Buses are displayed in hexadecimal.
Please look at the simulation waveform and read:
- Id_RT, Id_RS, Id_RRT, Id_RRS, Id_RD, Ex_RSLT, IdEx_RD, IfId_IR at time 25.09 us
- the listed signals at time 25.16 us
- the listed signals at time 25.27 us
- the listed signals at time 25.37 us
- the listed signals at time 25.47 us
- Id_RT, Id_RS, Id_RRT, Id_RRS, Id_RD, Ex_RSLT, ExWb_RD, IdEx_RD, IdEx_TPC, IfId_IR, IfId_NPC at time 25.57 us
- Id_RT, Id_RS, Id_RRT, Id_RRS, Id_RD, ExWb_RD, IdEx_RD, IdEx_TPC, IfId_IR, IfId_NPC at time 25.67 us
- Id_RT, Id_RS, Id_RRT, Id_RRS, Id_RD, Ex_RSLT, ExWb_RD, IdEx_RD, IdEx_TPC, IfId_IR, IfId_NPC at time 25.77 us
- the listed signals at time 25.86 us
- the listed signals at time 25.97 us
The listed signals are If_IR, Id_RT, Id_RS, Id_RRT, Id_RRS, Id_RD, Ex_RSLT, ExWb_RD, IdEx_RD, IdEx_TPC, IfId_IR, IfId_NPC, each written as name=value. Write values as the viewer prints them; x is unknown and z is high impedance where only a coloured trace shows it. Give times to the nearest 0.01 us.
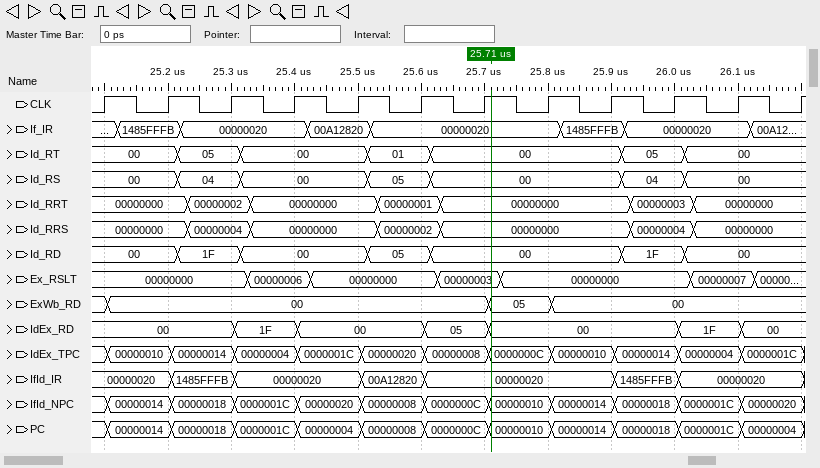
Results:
Id_RT=00, Id_RS=00, Id_RRT=00000000, Id_RRS=00000000, Id_RD=00, Ex_RSLT=00000000, IdEx_RD=00, IfId_IR=00000020
If_IR=1485FFFB, Id_RT=00, Id_RS=00, Id_RRT=00000000, Id_RRS=00000000, Id_RD=00, Ex_RSLT=00000000, ExWb_RD=00, IdEx_RD=00, IdEx_TPC=00000010, IfId_IR=00000020, IfId_NPC=00000014
If_IR=00000020, Id_RT=05, Id_RS=04, Id_RRT=00000002, Id_RRS=00000004, Id_RD=1F, Ex_RSLT=00000000, ExWb_RD=00, IdEx_RD=00, IdEx_TPC=00000014, IfId_IR=1485FFFB, IfId_NPC=00000018
If_IR=00000020, Id_RT=00, Id_RS=00, Id_RRT=00000000, Id_RRS=00000000, Id_RD=00, Ex_RSLT=00000006, ExWb_RD=00, IdEx_RD=1F, IdEx_TPC=00000004, IfId_IR=00000020, IfId_NPC=0000001C
If_IR=00A12820, Id_RT=00, Id_RS=00, Id_RRT=00000000, Id_RRS=00000000, Id_RD=00, Ex_RSLT=00000000, ExWb_RD=00, IdEx_RD=00, IdEx_TPC=0000001C, IfId_IR=00000020, IfId_NPC=00000020
Id_RT=01, Id_RS=05, Id_RRT=00000001, Id_RRS=00000002, Id_RD=05, Ex_RSLT=00000000, ExWb_RD=00, IdEx_RD=00, IdEx_TPC=00000020, IfId_IR=00A12820, IfId_NPC=00000008
Id_RT=00, Id_RS=00, Id_RRT=00000000, Id_RRS=00000000, Id_RD=00, ExWb_RD=00, IdEx_RD=05, IdEx_TPC=00000008, IfId_IR=00000020, IfId_NPC=0000000C
Id_RT=00, Id_RS=00, Id_RRT=00000000, Id_RRS=00000000, Id_RD=00, Ex_RSLT=00000000, ExWb_RD=05, IdEx_RD=00, IdEx_TPC=0000000C, IfId_IR=00000020, IfId_NPC=00000010
If_IR=1485FFFB, Id_RT=00, Id_RS=00, Id_RRT=00000000, Id_RRS=00000000, Id_RD=00, Ex_RSLT=00000000, ExWb_RD=00, IdEx_RD=00, IdEx_TPC=00000010, IfId_IR=00000020, IfId_NPC=00000014
If_IR=00000020, Id_RT=05, Id_RS=04, Id_RRT=00000003, Id_RRS=00000004, Id_RD=1F, Ex_RSLT=00000000, ExWb_RD=00, IdEx_RD=00, IdEx_TPC=00000014, IfId_IR=1485FFFB, IfId_NPC=00000018
